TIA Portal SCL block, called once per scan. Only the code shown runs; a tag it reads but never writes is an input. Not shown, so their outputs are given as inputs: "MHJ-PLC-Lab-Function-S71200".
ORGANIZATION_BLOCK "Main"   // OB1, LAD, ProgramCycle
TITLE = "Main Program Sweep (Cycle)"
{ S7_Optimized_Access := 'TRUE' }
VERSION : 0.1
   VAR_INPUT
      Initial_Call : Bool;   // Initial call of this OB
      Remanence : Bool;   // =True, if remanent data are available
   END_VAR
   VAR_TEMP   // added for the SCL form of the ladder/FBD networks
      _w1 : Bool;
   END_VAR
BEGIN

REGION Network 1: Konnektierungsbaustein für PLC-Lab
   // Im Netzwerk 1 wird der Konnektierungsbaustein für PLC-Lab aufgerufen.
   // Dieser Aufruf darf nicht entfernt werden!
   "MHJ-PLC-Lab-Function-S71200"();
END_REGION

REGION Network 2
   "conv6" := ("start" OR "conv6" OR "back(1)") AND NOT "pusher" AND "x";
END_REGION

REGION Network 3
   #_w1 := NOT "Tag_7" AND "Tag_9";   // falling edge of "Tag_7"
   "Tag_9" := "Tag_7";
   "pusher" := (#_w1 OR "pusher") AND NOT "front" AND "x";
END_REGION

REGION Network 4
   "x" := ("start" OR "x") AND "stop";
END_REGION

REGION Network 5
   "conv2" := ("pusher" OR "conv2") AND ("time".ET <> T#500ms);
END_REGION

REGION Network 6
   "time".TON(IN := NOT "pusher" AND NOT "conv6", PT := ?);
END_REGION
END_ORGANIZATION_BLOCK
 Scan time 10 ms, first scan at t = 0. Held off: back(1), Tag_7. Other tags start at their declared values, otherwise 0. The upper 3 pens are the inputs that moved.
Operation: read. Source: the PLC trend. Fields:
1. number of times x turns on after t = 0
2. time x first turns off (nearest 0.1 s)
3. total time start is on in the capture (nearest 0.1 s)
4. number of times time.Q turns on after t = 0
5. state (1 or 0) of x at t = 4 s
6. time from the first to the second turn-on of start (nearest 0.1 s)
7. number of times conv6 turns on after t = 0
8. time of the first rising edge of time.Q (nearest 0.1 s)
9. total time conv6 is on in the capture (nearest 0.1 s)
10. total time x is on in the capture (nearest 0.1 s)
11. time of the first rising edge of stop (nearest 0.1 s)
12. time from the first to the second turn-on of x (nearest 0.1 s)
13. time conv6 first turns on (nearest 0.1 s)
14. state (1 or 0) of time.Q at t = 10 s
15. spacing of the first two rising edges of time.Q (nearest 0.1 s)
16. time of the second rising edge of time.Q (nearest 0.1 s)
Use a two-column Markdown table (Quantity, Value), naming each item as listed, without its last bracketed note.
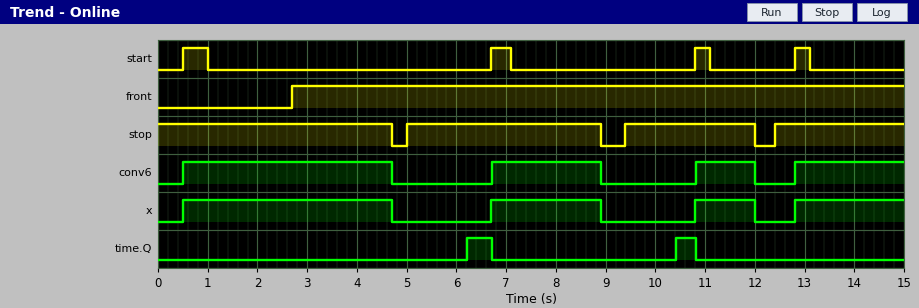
| Quantity | Value |
|---|---|
| number of times x turns on after t = 0 | 4 |
| time x first turns off | 4.7 s |
| total time start is on in the capture | 1.5 s |
| number of times time.Q turns on after t = 0 | 2 |
| state (1 or 0) of x at t = 4 s | 1 |
| time from the first to the second turn-on of start | 6.2 s |
| number of times conv6 turns on after t = 0 | 4 |
| time of the first rising edge of time.Q | 6.2 s |
| total time conv6 is on in the capture | 9.8 s |
| total time x is on in the capture | 9.8 s |
| time of the first rising edge of stop | 5.0 s |
| time from the first to the second turn-on of x | 6.2 s |
| time conv6 first turns on | 0.5 s |
| state (1 or 0) of time.Q at t = 10 s | 0 |
| spacing of the first two rising edges of time.Q | 4.2 s |
| time of the second rising edge of time.Q | 10.4 s |
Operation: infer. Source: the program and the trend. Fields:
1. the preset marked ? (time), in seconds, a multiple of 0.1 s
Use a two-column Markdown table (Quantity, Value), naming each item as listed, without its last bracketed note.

| Quantity | Value |
|---|---|
| the preset marked ? (time), in seconds, a multiple of 0.1 s | 1.5 s |
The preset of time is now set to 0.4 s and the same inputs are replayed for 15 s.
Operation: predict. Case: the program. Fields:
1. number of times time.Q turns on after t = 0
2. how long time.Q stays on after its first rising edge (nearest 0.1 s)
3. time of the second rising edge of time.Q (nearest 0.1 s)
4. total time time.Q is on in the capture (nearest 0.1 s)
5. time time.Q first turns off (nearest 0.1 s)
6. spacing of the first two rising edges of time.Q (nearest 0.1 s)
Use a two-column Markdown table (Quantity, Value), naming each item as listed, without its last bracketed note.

| Quantity | Value |
|---|---|
| number of times time.Q turns on after t = 0 | 4 |
| how long time.Q stays on after its first rising edge | 0.1 s |
| time of the second rising edge of time.Q | 5.1 s |
| total time time.Q is on in the capture | 3.6 s |
| time time.Q first turns off | 0.5 s |
| spacing of the first two rising edges of time.Q | 4.7 s |
